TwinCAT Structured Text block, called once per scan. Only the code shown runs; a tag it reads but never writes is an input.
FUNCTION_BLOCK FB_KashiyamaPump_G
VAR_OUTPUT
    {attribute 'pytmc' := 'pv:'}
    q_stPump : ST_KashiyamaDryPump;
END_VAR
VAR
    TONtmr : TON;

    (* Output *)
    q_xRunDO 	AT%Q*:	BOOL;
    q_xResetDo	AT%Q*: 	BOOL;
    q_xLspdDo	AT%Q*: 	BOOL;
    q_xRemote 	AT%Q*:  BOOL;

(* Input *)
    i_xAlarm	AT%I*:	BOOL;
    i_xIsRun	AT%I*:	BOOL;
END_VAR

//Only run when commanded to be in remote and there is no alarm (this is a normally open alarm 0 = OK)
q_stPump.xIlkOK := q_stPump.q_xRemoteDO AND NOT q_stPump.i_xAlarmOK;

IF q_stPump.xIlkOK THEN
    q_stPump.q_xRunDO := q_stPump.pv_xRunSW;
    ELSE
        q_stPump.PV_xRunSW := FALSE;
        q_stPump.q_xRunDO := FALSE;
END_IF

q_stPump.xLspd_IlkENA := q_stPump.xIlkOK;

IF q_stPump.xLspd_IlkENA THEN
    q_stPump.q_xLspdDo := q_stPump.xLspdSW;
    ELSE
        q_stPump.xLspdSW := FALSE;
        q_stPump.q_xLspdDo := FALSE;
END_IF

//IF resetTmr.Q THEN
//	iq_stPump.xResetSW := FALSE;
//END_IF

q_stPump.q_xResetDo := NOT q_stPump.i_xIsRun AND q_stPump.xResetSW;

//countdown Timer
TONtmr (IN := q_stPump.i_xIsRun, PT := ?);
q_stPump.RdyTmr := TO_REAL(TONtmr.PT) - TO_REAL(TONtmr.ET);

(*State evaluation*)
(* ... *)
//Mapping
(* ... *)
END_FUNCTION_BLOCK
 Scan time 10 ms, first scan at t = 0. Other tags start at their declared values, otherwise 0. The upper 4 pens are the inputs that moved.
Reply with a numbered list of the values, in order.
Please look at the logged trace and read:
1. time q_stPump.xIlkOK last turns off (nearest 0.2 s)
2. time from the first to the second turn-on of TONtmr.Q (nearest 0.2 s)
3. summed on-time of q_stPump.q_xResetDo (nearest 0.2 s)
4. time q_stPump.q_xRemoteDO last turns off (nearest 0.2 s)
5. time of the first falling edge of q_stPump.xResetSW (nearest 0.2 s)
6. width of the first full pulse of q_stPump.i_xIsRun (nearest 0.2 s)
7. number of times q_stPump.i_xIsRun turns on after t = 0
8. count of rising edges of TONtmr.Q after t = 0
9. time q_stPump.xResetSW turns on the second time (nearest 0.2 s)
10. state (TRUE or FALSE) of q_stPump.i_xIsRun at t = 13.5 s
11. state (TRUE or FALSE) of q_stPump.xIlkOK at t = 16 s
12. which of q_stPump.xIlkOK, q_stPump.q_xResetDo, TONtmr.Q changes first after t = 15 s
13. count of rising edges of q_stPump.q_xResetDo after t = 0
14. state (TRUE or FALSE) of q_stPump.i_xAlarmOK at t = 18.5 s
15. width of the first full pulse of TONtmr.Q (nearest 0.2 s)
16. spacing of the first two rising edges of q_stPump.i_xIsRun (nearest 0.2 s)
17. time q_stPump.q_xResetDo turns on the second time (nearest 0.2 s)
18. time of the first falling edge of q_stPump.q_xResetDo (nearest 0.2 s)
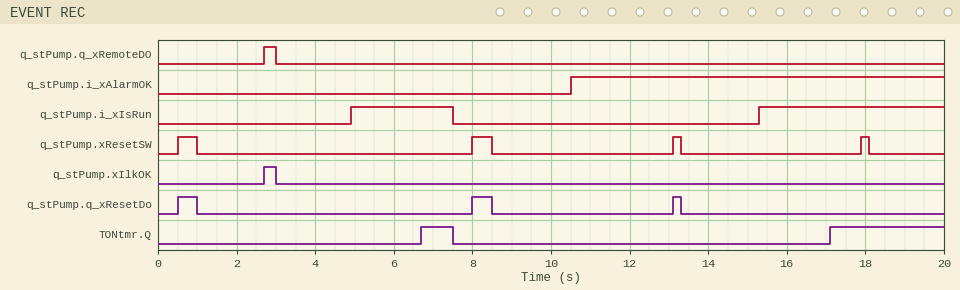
1. 3.0 s
2. 10.4 s
3. 1.2 s
4. 3.0 s
5. 1.0 s
6. 2.6 s
7. 2
8. 2
9. 8.0 s
10. FALSE
11. FALSE
12. TONtmr.Q
13. 3
14. TRUE
15. 0.8 s
16. 10.4 s
17. 8.0 s
18. 1.0 s
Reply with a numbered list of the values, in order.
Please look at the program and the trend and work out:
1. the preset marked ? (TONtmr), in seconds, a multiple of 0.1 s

1. 1.8 s
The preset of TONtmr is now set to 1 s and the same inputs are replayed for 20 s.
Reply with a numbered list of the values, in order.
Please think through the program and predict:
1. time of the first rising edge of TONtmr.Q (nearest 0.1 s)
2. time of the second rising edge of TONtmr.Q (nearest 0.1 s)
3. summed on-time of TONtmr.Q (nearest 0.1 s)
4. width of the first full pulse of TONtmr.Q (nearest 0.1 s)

1. 5.9 s
2. 16.3 s
3. 5.3 s
4. 1.6 s
